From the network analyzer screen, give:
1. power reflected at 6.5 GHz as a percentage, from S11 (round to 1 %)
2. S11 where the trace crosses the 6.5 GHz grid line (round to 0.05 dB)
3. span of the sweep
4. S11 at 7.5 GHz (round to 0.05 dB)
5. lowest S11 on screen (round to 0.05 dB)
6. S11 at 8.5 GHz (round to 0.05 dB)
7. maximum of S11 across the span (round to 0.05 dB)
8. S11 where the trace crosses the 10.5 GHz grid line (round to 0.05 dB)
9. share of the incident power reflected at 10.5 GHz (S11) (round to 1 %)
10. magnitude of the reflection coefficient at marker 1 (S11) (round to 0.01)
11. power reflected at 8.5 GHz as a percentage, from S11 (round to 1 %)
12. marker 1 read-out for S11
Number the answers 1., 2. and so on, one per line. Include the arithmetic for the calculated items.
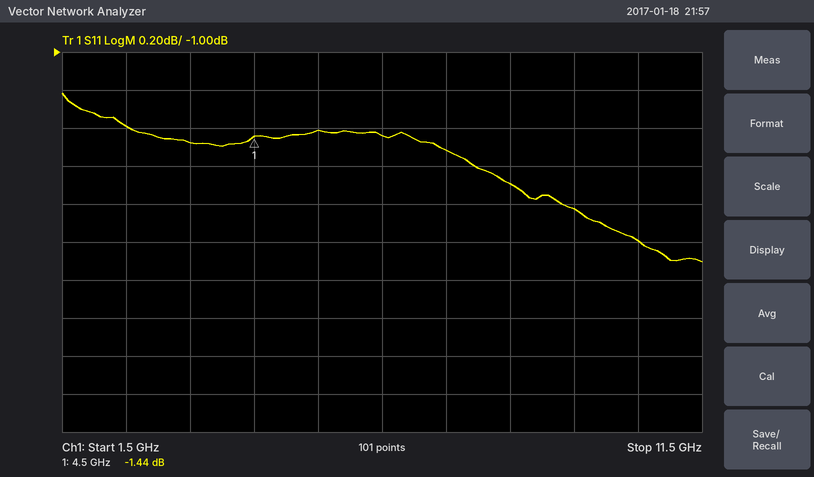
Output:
1. 10^(-1.45/10) ≈ 72 %
2. -1.45 dB
3. 10 GHz
4. -1.50 dB
5. -2.10 dB
6. -1.70 dB
7. -1.20 dB
8. -2.00 dB
9. 10^(-2/10) ≈ 63 %
10. 10^(-1.44/20) ≈ 0.85
11. 10^(-1.7/10) ≈ 68 %
12. -1.44 dB
